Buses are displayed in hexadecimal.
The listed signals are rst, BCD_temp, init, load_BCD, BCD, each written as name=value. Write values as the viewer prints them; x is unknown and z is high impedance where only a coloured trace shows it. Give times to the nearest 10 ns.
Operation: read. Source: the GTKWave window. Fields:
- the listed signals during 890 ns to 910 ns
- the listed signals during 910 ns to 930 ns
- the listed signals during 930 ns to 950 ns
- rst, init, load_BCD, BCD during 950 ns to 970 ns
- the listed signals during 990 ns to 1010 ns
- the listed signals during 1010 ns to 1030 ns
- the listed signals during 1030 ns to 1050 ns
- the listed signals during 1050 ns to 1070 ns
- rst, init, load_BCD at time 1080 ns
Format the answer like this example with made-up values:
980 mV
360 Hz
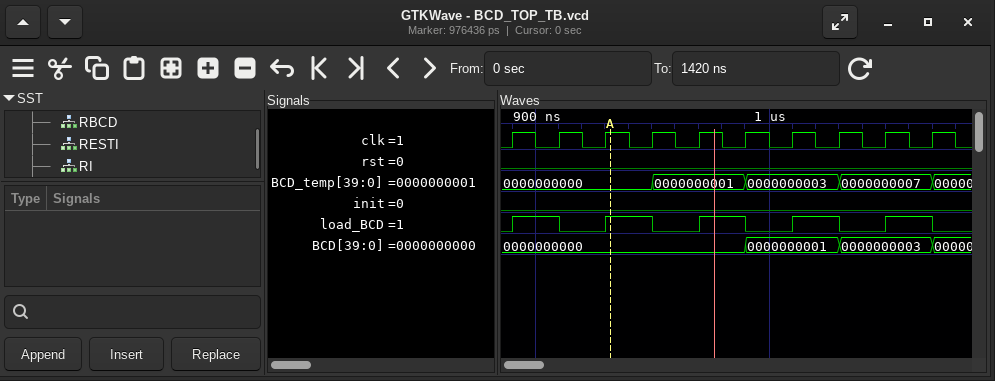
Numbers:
rst=0, BCD_temp=0000000000, init=0, load_BCD=1, BCD=0000000000
rst=0, BCD_temp=0000000000, init=0, load_BCD=0, BCD=0000000000
rst=0, BCD_temp=0000000000, init=0, load_BCD=1, BCD=0000000000
rst=0, init=0, load_BCD=0, BCD=0000000000
rst=0, BCD_temp=0000000003, init=0, load_BCD=0, BCD=0000000001
rst=0, BCD_temp=0000000003, init=0, load_BCD=1, BCD=0000000001
rst=0, BCD_temp=0000000007, init=0, load_BCD=0, BCD=0000000003
rst=0, BCD_temp=0000000007, init=0, load_BCD=1, BCD=0000000003
rst=0, init=0, load_BCD=0
